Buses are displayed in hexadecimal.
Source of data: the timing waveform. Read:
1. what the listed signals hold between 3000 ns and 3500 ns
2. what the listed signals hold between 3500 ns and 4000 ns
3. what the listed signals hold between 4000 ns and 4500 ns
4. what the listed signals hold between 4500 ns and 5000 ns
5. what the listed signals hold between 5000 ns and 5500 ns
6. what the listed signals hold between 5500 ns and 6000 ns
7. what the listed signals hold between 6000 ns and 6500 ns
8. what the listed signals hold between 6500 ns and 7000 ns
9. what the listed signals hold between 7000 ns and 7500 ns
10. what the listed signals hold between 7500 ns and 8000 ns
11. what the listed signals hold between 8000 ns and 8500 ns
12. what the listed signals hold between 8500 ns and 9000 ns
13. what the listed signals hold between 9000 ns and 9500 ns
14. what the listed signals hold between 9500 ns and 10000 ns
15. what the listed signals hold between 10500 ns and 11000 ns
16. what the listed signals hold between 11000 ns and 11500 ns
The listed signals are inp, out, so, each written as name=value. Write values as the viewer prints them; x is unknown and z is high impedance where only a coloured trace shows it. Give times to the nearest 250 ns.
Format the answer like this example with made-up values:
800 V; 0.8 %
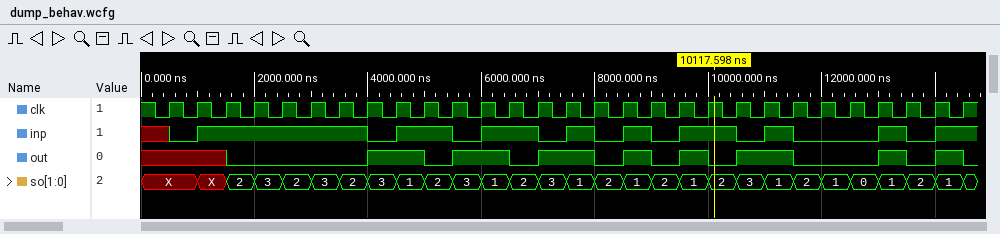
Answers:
inp=1, out=0, so=3; inp=1, out=0, so=2; inp=0, out=1, so=3; inp=1, out=1, so=1; inp=1, out=0, so=2; inp=0, out=1, so=3; inp=1, out=1, so=1; inp=1, out=0, so=2; inp=0, out=1, so=3; inp=1, out=1, so=1; inp=0, out=0, so=2; inp=1, out=1, so=1; inp=0, out=0, so=2; inp=1, out=1, so=1; inp=0, out=1, so=3; inp=1, out=1, so=1
